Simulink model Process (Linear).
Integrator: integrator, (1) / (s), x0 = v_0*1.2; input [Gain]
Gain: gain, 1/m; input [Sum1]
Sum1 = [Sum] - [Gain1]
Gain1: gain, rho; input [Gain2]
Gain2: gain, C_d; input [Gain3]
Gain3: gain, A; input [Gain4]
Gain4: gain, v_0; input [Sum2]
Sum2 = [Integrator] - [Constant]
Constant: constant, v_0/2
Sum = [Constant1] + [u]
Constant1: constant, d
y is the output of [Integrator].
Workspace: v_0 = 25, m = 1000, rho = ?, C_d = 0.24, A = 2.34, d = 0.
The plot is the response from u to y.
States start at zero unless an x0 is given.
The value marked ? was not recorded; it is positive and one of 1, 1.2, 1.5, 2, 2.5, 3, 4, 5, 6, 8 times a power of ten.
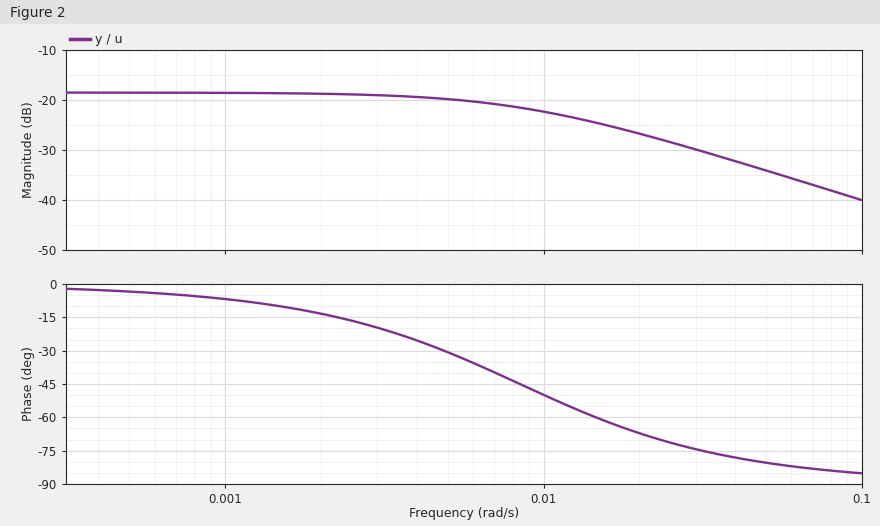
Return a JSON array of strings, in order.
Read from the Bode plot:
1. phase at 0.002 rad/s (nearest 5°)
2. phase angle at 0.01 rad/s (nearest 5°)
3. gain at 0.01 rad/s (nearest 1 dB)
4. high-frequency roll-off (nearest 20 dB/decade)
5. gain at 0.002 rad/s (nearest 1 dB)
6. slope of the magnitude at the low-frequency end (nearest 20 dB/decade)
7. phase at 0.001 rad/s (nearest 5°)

["-15°", "-50°", "-22 dB", "-20 dB/decade", "-19 dB", "0 dB/decade", "-5°"]
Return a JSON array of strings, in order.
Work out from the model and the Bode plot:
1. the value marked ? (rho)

["0.6"]
